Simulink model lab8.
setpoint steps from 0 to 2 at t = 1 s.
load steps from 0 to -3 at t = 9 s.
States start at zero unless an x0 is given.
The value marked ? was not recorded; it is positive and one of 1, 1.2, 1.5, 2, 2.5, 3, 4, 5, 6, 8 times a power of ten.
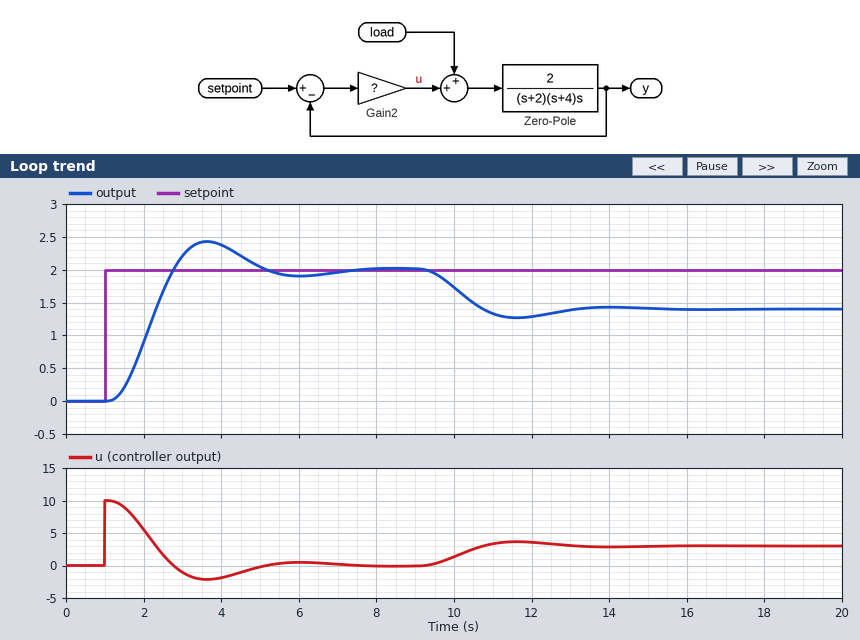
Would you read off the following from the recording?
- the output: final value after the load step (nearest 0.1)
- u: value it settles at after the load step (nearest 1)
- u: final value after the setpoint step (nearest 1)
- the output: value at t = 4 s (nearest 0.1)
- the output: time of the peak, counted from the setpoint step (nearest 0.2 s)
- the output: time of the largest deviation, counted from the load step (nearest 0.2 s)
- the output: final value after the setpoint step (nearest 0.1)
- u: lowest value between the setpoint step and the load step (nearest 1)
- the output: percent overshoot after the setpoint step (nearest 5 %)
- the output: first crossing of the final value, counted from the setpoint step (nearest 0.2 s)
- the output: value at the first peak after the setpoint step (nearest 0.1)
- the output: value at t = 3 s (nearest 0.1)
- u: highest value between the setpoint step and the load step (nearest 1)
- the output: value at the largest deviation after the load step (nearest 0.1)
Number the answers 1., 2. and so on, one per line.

1. 1.4
2. 3
3. 0
4. 2.4
5. 2.6 s
6. 2.6 s
7. 2.0
8. -2
9. 20 %
10. 1.8 s
11. 2.4
12. 2.2
13. 10
14. 1.3
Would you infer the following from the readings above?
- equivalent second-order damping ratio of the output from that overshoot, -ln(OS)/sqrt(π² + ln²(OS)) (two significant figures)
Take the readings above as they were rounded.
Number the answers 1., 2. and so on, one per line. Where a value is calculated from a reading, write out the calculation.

1. ln(0.2) = -1.609; 1.609 / sqrt(9.870 + 2.590) = 0.46
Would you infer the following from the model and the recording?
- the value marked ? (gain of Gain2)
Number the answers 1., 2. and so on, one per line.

1. 5
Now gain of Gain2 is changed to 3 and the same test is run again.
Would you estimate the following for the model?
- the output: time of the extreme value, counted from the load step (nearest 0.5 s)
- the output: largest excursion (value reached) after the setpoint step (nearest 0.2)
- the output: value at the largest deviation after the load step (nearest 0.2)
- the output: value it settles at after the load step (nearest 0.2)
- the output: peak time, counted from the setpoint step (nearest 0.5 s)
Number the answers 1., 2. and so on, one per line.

1. 4.0 s
2. 2.2
3. 1.0
4. 1.0
5. 4.0 s
